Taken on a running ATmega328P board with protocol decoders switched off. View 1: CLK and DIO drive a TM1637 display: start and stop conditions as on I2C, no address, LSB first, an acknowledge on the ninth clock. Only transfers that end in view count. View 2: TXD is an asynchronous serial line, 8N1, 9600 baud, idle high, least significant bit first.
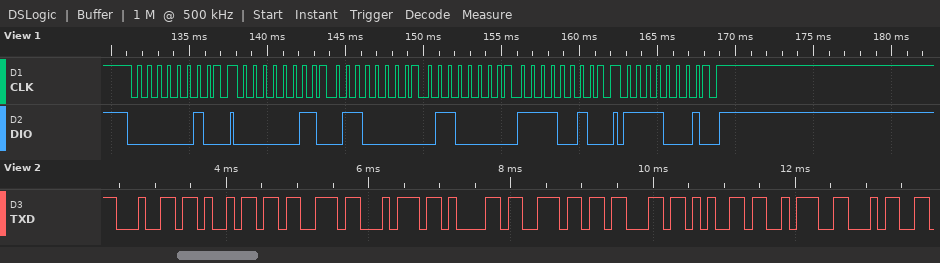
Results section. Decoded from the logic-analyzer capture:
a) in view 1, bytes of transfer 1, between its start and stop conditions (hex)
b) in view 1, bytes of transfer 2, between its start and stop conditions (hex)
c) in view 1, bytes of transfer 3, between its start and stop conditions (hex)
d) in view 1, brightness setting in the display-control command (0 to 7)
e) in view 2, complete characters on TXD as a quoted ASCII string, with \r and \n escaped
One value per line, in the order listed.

40
C0 06 06 4F
8F
7
"distance:4"
